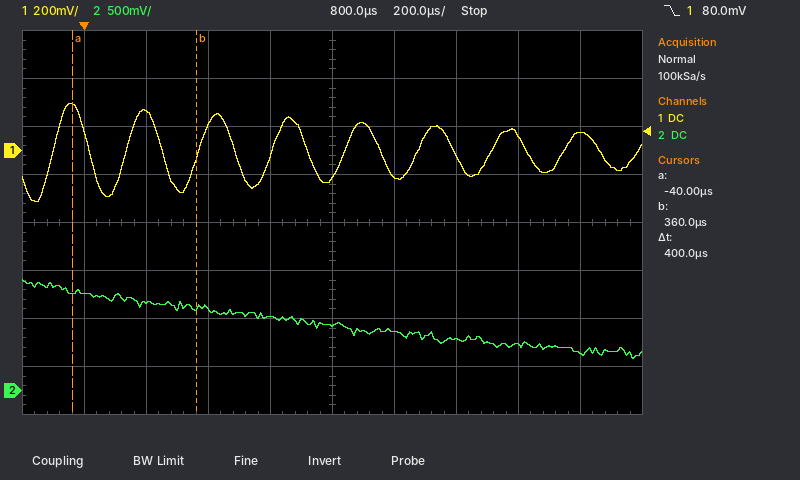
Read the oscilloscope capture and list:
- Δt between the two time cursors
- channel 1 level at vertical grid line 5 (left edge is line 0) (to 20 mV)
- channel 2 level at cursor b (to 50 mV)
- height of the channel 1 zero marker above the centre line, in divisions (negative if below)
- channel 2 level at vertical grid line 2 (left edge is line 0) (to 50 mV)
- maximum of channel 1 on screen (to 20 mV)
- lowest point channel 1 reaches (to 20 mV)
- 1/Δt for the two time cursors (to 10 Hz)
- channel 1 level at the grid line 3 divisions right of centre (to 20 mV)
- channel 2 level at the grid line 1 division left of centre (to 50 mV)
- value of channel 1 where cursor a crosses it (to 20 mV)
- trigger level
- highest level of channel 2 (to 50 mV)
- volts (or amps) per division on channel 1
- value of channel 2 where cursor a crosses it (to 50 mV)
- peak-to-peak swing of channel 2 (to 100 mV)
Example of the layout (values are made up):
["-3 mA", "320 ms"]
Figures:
["400 µs", "-120 mV", "850 mV", "+1.5 div", "900 mV", "200 mV", "-220 mV", "2.50 kHz", "60 mV", "750 mV", "180 mV", "80.0 mV", "1.15 V", "200 mV", "1.00 V", "800 mV"]
